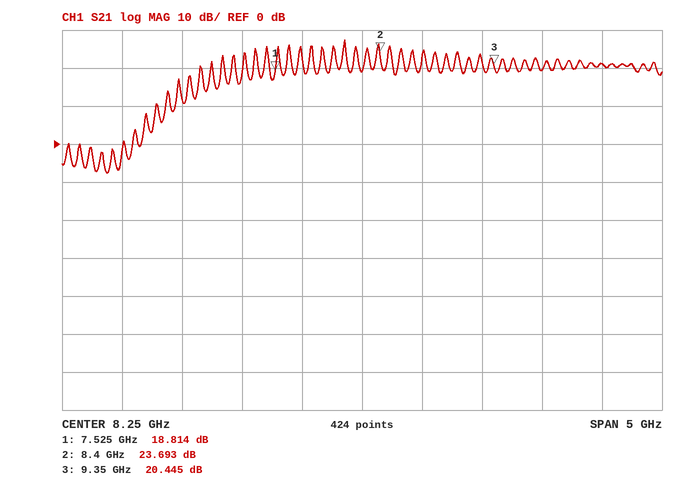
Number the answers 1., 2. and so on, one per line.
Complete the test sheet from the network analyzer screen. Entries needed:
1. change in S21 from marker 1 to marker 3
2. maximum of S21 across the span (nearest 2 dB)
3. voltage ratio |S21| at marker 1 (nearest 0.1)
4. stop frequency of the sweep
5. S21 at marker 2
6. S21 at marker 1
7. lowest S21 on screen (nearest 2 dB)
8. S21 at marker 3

1. 1.631 dB
2. 28 dB
3. 8.7
4. 10.75 GHz
5. 23.693 dB
6. 18.814 dB
7. -8 dB
8. 20.445 dB
